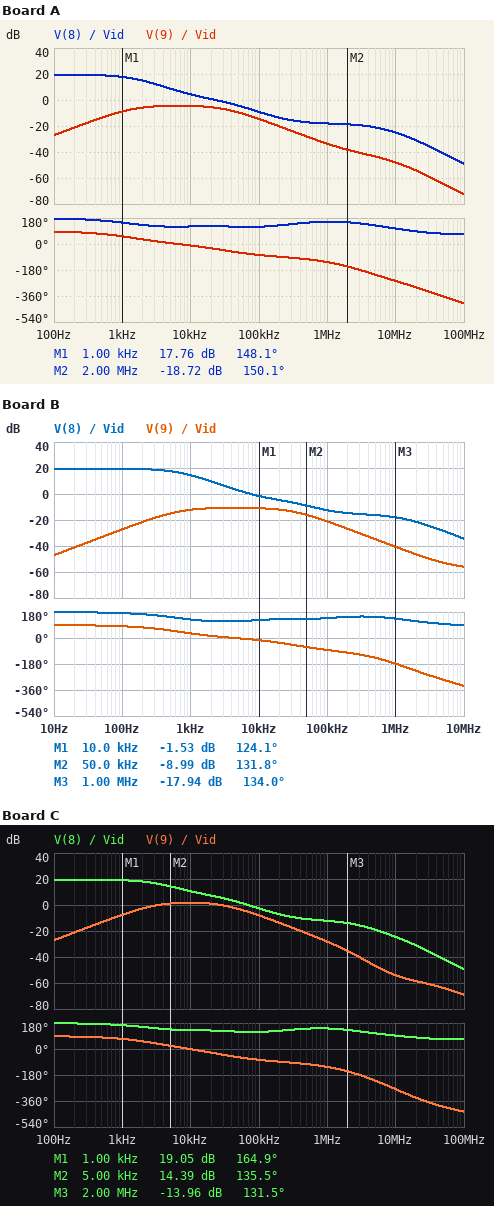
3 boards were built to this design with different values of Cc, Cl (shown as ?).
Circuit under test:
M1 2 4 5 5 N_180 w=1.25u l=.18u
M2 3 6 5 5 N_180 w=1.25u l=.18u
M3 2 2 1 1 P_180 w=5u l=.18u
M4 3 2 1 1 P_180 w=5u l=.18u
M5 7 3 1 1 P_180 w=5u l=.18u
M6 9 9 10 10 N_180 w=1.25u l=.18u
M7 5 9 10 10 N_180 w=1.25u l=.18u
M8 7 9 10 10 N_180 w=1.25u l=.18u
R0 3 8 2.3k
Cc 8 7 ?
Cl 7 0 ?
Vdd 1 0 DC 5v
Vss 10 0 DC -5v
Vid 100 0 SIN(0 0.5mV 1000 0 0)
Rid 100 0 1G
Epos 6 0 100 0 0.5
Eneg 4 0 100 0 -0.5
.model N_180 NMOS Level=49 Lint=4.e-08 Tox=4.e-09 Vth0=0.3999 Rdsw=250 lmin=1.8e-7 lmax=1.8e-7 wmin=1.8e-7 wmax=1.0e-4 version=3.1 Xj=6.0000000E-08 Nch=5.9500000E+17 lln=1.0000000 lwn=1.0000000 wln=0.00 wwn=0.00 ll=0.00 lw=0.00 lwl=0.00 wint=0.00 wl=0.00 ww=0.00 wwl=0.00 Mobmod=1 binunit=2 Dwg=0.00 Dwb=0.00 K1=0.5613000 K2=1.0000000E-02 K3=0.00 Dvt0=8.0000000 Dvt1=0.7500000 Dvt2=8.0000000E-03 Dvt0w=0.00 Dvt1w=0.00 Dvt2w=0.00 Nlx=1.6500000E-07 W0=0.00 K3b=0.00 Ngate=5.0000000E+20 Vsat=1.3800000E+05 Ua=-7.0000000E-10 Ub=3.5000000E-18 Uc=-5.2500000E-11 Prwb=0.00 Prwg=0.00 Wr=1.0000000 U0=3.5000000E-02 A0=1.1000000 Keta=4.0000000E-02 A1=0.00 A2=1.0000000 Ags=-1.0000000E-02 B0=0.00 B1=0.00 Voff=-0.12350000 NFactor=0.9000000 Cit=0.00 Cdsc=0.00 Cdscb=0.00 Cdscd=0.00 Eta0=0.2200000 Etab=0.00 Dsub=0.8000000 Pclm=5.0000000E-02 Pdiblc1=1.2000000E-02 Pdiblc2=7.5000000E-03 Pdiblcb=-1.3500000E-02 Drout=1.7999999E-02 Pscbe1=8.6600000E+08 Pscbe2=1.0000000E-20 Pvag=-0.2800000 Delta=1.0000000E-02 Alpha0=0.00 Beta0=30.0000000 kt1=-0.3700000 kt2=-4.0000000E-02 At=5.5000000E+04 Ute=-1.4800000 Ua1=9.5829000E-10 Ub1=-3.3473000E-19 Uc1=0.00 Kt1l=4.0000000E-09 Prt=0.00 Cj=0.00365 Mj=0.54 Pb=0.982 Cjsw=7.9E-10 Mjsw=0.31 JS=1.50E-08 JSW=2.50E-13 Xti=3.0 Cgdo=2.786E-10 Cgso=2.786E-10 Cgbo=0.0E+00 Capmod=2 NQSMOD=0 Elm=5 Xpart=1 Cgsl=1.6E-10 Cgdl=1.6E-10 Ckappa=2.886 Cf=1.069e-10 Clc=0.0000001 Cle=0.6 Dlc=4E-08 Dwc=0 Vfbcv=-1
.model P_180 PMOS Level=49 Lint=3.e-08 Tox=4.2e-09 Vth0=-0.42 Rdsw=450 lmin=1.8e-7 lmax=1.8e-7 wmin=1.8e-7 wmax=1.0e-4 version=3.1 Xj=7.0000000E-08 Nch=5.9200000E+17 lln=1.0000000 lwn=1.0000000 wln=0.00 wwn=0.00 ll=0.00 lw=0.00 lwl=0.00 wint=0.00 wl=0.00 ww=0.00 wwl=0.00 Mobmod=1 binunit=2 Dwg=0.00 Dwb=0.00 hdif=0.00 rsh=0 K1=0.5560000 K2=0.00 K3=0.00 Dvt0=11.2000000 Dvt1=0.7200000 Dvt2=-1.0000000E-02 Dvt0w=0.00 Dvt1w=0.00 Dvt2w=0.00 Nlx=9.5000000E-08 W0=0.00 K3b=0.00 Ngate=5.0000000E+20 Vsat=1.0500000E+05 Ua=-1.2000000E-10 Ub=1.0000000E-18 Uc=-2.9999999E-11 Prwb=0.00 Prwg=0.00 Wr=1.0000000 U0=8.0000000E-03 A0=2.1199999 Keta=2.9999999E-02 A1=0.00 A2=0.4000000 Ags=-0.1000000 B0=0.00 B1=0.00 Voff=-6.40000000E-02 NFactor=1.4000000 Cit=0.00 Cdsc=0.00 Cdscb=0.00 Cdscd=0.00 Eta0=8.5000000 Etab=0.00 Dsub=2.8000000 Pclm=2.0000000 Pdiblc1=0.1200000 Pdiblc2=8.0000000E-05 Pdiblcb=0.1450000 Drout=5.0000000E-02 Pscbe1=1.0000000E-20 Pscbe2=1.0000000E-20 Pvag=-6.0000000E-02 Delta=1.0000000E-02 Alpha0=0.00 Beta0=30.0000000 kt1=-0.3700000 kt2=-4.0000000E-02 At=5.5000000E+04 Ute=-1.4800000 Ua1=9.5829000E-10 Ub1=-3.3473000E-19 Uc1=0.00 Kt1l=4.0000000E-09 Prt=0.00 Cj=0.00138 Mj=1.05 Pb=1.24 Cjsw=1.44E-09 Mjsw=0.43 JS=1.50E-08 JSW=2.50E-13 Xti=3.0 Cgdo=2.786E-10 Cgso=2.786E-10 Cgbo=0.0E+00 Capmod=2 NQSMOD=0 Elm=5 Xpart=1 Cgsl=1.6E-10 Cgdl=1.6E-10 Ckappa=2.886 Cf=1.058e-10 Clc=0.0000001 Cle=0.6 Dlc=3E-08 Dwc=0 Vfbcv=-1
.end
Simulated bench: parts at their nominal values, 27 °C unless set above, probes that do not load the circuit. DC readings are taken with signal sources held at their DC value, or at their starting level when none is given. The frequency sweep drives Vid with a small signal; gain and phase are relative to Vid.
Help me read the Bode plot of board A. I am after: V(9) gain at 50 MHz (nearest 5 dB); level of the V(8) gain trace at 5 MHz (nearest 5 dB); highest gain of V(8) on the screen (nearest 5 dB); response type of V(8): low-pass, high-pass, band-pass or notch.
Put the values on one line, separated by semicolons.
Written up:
-65 dB; -20 dB; 20 dB; low-pass
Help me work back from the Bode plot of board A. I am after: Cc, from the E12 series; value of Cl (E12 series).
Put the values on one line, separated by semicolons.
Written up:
3.9 pF; 1.5 pF
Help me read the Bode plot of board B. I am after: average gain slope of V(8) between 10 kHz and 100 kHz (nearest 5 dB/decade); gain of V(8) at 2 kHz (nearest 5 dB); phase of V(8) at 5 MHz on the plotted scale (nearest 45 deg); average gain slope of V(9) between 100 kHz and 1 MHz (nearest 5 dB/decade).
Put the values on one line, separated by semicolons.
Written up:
-10 dB/decade; 10 dB; 90 deg; -20 dB/decade
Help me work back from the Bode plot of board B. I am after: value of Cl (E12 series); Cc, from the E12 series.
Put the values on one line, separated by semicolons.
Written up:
6.8 pF; 8.2 pF
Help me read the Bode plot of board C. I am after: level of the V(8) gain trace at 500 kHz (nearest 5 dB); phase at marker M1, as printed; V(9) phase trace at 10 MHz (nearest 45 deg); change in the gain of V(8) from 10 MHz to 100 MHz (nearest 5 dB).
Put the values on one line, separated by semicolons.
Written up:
-10 dB; 164.9 deg; -270 deg; -25 dB
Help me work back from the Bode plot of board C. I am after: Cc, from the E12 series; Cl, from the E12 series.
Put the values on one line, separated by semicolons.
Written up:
1.8 pF; 3.3 pF
